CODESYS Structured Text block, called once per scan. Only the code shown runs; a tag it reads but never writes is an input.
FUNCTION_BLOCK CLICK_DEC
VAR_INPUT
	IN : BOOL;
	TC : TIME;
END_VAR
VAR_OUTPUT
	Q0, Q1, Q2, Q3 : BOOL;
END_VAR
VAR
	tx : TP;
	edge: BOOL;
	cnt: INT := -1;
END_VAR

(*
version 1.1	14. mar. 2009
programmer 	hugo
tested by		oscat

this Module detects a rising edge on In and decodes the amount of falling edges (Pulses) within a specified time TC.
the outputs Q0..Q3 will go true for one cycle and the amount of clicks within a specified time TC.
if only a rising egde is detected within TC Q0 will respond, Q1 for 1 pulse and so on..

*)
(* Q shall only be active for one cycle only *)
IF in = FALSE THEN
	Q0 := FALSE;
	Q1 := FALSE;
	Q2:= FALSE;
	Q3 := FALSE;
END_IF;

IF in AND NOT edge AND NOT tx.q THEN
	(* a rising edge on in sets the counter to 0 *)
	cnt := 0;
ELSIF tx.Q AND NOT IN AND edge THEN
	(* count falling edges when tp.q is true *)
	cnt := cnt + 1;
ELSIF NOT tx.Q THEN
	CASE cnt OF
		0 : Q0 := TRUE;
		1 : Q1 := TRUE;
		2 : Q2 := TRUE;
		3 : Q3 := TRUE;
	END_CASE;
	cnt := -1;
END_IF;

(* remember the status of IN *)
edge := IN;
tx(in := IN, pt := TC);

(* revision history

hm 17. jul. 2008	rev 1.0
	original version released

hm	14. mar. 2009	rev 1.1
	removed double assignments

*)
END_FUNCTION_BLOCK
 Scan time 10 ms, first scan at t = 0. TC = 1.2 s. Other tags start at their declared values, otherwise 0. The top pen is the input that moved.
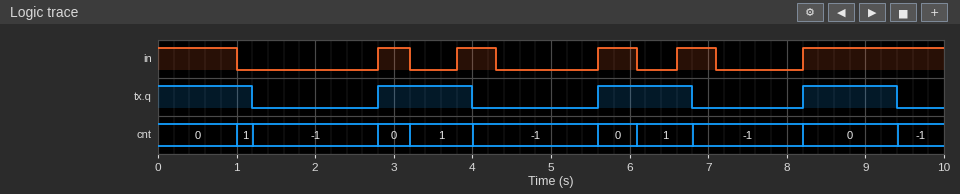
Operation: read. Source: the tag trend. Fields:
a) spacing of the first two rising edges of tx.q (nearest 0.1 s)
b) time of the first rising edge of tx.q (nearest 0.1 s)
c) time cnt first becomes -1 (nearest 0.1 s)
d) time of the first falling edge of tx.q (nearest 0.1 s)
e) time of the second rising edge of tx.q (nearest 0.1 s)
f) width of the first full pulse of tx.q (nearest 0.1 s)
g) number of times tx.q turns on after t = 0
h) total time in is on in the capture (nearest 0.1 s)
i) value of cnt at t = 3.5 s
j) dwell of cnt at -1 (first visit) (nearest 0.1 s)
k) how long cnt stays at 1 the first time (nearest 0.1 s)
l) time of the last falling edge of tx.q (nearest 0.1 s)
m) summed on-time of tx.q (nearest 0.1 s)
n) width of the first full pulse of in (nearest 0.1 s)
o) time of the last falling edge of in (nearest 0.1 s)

2.8 s
2.8 s
1.2 s
1.2 s
5.6 s
1.2 s
3
4.7 s
1
1.6 s
0.2 s
9.4 s
4.8 s
0.4 s
7.1 s
